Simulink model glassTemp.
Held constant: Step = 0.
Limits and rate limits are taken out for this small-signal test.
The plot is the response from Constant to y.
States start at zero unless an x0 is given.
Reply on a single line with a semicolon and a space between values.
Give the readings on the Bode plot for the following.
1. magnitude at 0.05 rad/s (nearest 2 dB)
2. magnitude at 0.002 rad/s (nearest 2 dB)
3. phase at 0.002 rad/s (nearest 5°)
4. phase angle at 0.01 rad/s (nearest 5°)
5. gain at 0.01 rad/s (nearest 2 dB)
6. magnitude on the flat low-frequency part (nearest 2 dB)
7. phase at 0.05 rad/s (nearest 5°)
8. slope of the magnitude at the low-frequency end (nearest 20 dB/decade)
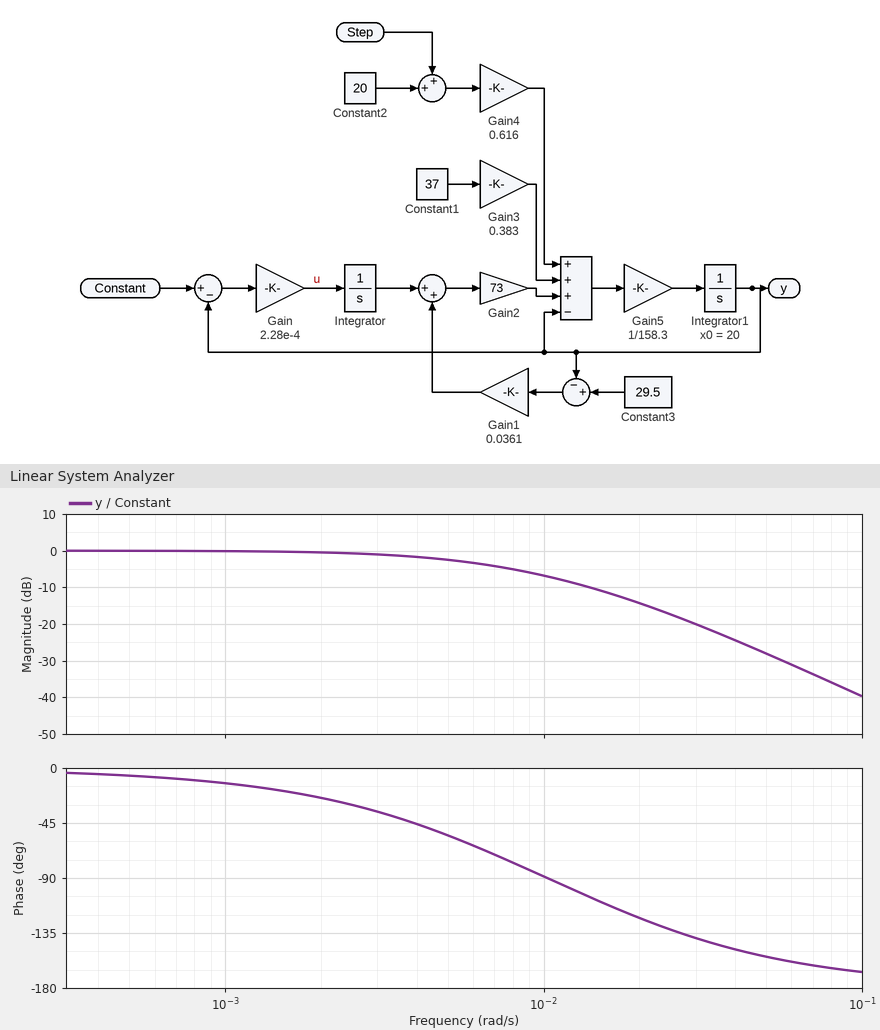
-28 dB; 0 dB; -25°; -90°; -6 dB; 0 dB; -155°; 0 dB/decade
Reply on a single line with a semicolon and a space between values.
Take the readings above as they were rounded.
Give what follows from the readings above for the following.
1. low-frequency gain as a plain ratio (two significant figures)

1.0
